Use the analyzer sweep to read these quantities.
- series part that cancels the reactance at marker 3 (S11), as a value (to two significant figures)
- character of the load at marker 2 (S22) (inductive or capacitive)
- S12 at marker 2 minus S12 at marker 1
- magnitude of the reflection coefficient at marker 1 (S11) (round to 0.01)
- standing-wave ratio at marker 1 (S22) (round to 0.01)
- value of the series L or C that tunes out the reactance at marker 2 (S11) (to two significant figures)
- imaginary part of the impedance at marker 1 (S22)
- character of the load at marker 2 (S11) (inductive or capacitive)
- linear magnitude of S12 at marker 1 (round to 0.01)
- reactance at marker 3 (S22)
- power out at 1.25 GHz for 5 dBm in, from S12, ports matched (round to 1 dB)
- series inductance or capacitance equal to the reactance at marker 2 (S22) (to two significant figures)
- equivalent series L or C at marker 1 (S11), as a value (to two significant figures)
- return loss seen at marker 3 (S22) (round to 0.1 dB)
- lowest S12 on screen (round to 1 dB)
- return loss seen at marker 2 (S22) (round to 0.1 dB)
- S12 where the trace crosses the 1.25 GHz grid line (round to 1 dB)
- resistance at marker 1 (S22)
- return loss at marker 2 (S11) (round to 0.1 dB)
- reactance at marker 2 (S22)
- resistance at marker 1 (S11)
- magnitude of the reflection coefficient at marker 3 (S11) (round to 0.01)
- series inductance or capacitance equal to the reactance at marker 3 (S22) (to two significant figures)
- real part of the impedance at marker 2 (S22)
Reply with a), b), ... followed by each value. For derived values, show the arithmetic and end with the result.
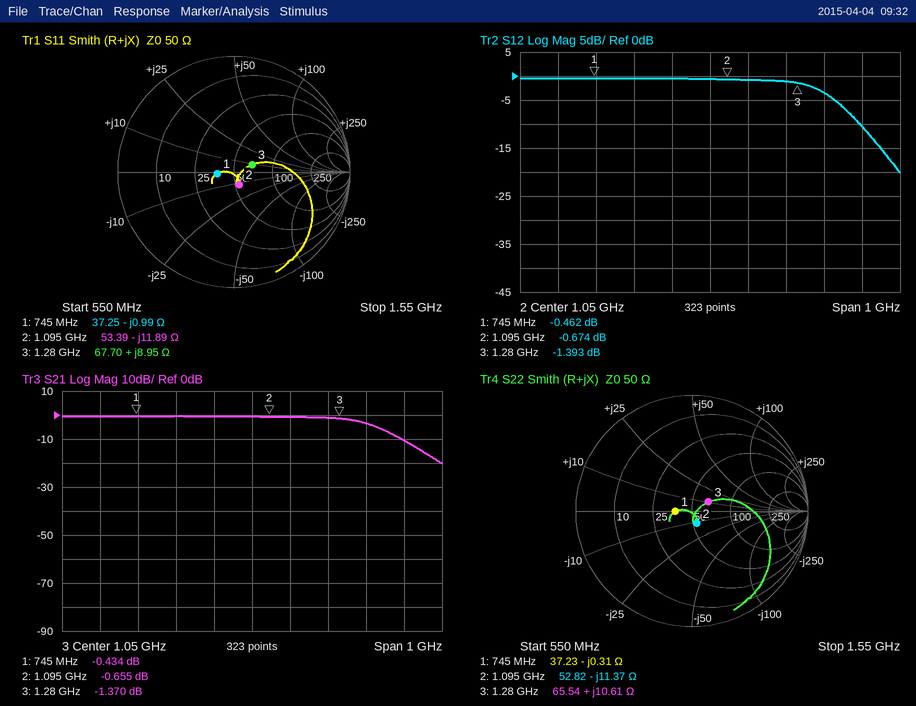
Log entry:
a) C = 1/(2π × 1.28 GHz × 8.95 Ω) ≈ 14 pF
b) capacitive
c) -0.674 − (-0.462) = -0.212 dB
d) 0.15
e) 1.34
f) L = 11.89 Ω/(2π × 1.095 GHz) ≈ 1.7 nH
g) -0.31 Ω
h) capacitive
i) 10^(-0.462/20) ≈ 0.95
j) +10.61 Ω
k) 5 dBm + (-1 dB) = 4 dBm
l) C = 1/(2π × 1.095 GHz × 11.37 Ω) ≈ 13 pF
m) C = 1/(2π × 745 MHz × 0.99 Ω) ≈ 216 pF, so 220 pF to two significant figures
n) 15.8 dB
o) -20 dB
p) 18.9 dB
q) -1 dB
r) 37.23 Ω
s) 18.5 dB
t) -11.37 Ω
u) 37.25 Ω
v) 0.17
w) L = 10.61 Ω/(2π × 1.28 GHz) ≈ 1.3 nH
x) 52.82 Ω
